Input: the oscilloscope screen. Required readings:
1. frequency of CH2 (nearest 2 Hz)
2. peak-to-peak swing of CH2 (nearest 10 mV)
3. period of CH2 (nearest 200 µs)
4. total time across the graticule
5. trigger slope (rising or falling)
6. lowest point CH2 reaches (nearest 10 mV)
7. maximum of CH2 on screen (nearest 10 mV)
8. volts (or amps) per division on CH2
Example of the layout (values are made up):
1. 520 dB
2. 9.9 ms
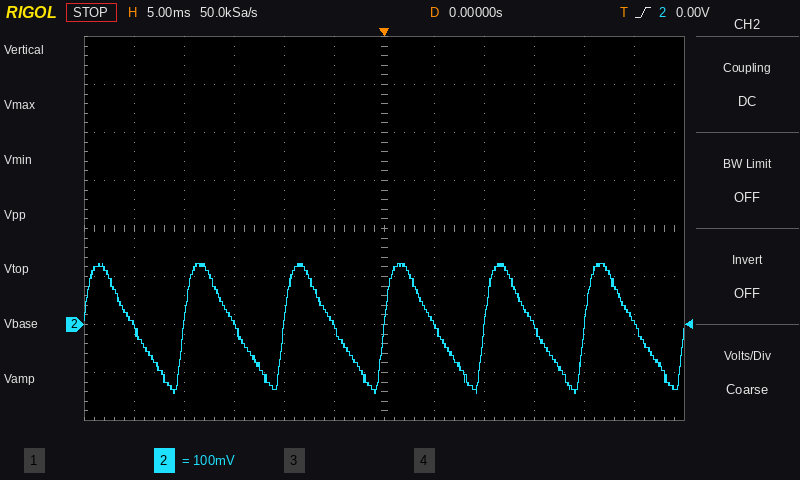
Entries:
1. 100 Hz
2. 270 mV
3. 10.0 ms
4. 60 ms
5. rising
6. -140 mV
7. 130 mV
8. 100 mV
